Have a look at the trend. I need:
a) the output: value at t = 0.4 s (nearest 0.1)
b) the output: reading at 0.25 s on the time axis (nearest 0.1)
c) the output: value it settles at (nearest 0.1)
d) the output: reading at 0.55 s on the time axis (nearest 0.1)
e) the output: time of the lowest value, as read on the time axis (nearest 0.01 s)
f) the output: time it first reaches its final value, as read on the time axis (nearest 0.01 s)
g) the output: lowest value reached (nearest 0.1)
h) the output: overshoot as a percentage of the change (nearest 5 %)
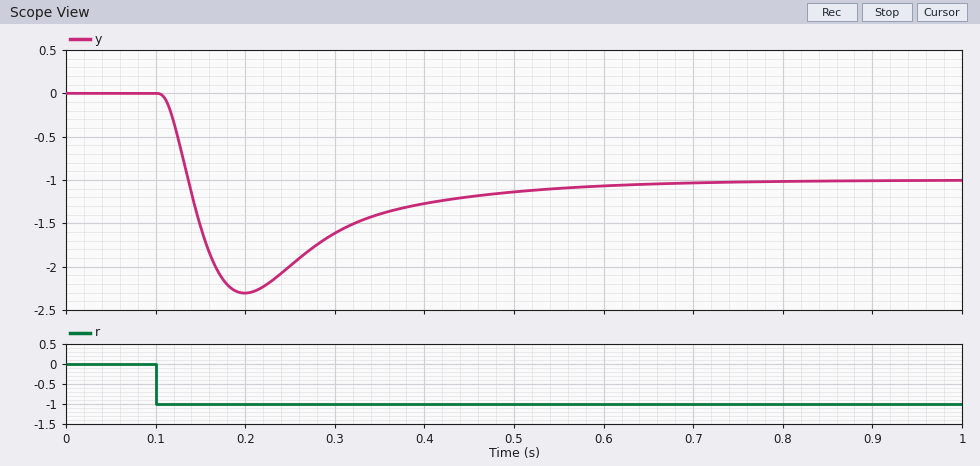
-1.3
-2.0
-1.0
-1.1
0.20 s
0.14 s
-2.3
130 %
